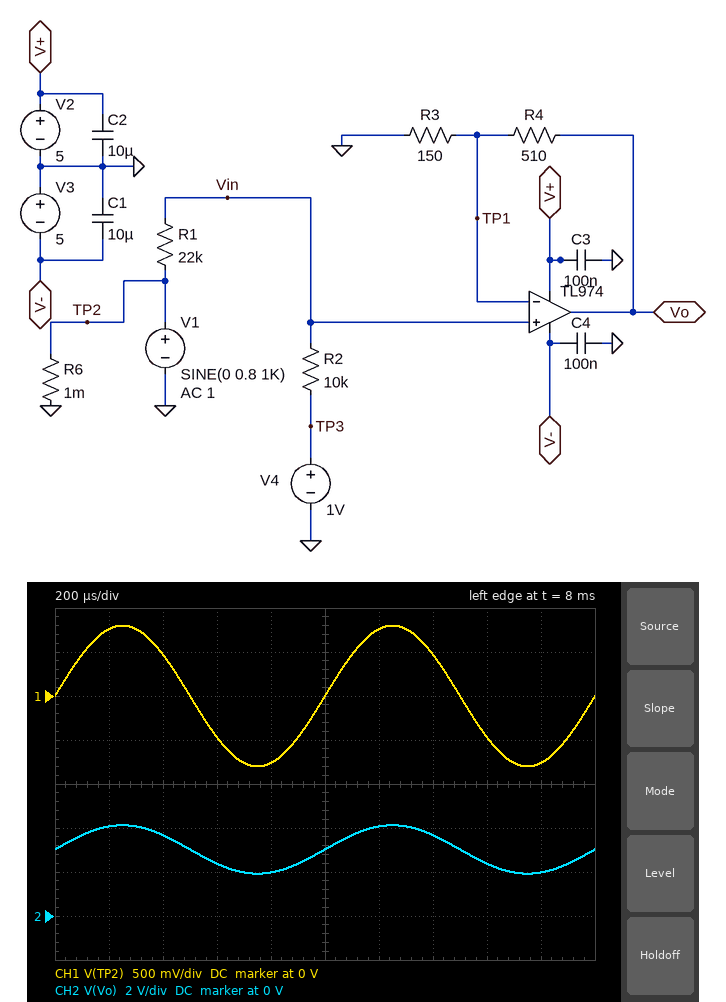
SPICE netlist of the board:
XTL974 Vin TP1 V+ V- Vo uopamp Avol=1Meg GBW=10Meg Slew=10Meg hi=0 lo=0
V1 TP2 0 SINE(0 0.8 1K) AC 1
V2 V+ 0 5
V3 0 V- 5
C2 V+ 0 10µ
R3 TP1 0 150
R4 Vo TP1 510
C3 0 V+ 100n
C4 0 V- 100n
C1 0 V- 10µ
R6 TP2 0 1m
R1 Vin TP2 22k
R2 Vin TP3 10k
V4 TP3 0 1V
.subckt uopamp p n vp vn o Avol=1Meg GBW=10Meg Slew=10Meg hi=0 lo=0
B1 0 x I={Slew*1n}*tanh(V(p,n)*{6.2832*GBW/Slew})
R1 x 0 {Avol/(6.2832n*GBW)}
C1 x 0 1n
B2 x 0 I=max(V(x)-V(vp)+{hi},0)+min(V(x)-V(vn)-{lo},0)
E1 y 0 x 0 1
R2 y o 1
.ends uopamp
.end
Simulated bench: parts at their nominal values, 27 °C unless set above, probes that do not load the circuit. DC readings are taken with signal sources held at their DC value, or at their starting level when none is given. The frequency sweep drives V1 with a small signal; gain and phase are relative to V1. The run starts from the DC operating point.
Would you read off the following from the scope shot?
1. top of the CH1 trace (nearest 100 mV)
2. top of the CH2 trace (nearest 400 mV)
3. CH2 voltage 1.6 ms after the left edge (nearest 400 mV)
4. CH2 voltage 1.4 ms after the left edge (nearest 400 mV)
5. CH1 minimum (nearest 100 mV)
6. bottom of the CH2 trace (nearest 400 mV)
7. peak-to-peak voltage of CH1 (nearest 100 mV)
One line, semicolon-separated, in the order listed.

800 mV; 4.0 V; 2.4 V; 3.6 V; -800 mV; 2.0 V; 1.6 V
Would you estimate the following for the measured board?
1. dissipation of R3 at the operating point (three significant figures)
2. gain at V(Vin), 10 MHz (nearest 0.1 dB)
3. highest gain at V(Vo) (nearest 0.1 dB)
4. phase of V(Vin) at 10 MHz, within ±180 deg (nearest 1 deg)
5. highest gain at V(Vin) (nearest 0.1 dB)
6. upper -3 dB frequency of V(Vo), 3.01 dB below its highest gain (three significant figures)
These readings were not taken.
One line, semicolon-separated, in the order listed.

3.15 mW; -10.1 dB; 2.8 dB; 0 deg; -10.1 dB; 2.27 MHz
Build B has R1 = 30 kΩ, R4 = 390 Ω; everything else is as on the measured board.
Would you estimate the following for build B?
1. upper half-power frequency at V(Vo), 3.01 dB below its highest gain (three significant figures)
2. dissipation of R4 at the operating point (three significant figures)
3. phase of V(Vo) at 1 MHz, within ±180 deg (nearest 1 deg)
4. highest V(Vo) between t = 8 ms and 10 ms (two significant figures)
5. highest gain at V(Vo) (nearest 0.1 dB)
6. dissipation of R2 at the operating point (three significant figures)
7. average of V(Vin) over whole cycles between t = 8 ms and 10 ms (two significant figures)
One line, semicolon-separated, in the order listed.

2.77 MHz; 9.75 mW; -20 deg; 3.4 V; -0.9 dB; 6.25 µW; 750 mV
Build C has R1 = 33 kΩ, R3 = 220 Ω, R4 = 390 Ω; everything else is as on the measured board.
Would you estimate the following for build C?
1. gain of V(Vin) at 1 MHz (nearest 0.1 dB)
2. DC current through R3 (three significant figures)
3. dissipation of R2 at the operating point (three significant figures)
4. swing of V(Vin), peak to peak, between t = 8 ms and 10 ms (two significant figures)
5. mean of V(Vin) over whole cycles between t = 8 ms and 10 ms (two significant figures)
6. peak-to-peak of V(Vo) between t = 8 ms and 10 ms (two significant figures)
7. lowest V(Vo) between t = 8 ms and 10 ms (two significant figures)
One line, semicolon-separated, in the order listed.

-12.7 dB; 3.49 mA; 5.41 µW; 370 mV; 770 mV; 1.0 V; 1.6 V
